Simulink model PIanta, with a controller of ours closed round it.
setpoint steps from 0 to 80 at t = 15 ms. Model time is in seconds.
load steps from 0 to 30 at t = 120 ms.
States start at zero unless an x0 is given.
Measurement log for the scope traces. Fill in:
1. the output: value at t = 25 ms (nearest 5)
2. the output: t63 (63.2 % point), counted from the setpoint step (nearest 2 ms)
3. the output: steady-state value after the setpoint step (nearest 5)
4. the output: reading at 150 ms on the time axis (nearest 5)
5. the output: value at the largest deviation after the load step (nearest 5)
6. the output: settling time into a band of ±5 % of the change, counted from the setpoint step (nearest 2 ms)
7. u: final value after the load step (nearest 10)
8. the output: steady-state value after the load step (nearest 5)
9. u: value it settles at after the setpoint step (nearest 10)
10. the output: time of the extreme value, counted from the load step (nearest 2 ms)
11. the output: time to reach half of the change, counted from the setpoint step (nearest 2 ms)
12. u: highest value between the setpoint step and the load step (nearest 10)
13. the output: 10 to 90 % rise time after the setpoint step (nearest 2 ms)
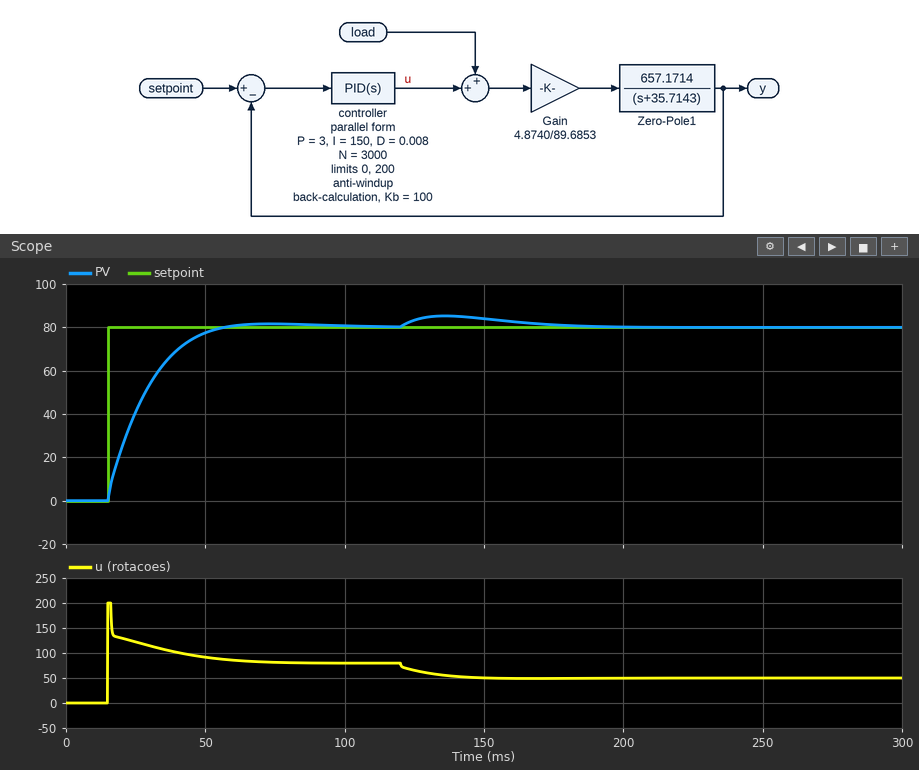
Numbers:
40
14 ms
80
85
85
32 ms
50
80
80
16 ms
10 ms
200
26 ms
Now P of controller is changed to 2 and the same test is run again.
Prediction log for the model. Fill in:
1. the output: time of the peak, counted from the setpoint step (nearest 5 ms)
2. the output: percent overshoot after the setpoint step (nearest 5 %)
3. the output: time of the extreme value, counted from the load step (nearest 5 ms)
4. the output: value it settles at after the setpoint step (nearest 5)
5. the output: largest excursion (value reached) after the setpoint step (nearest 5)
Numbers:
50 ms
10 %
20 ms
80
85
